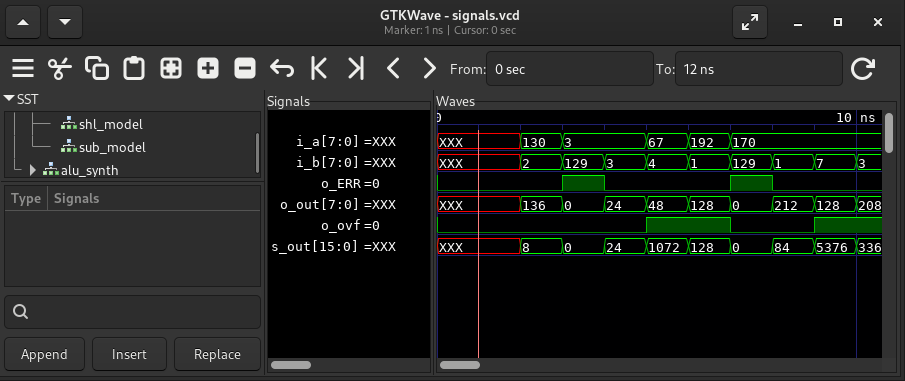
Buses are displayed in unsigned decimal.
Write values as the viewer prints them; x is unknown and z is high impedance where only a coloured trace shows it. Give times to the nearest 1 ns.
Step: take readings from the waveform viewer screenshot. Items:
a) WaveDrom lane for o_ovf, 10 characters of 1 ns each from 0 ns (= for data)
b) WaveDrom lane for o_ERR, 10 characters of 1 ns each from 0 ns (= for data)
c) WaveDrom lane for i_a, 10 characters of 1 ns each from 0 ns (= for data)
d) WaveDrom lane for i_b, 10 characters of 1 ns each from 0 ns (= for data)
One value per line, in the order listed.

{name: 'o_ovf', wave: '0....1.0.1'}
{name: 'o_ERR', wave: '0..10..10.'}
{name: 'i_a', wave: 'x.==.===..', data: '130 3 67 192 170'}
{name: 'i_b', wave: 'x.========', data: '2 129 3 4 1 129 1 7'}
